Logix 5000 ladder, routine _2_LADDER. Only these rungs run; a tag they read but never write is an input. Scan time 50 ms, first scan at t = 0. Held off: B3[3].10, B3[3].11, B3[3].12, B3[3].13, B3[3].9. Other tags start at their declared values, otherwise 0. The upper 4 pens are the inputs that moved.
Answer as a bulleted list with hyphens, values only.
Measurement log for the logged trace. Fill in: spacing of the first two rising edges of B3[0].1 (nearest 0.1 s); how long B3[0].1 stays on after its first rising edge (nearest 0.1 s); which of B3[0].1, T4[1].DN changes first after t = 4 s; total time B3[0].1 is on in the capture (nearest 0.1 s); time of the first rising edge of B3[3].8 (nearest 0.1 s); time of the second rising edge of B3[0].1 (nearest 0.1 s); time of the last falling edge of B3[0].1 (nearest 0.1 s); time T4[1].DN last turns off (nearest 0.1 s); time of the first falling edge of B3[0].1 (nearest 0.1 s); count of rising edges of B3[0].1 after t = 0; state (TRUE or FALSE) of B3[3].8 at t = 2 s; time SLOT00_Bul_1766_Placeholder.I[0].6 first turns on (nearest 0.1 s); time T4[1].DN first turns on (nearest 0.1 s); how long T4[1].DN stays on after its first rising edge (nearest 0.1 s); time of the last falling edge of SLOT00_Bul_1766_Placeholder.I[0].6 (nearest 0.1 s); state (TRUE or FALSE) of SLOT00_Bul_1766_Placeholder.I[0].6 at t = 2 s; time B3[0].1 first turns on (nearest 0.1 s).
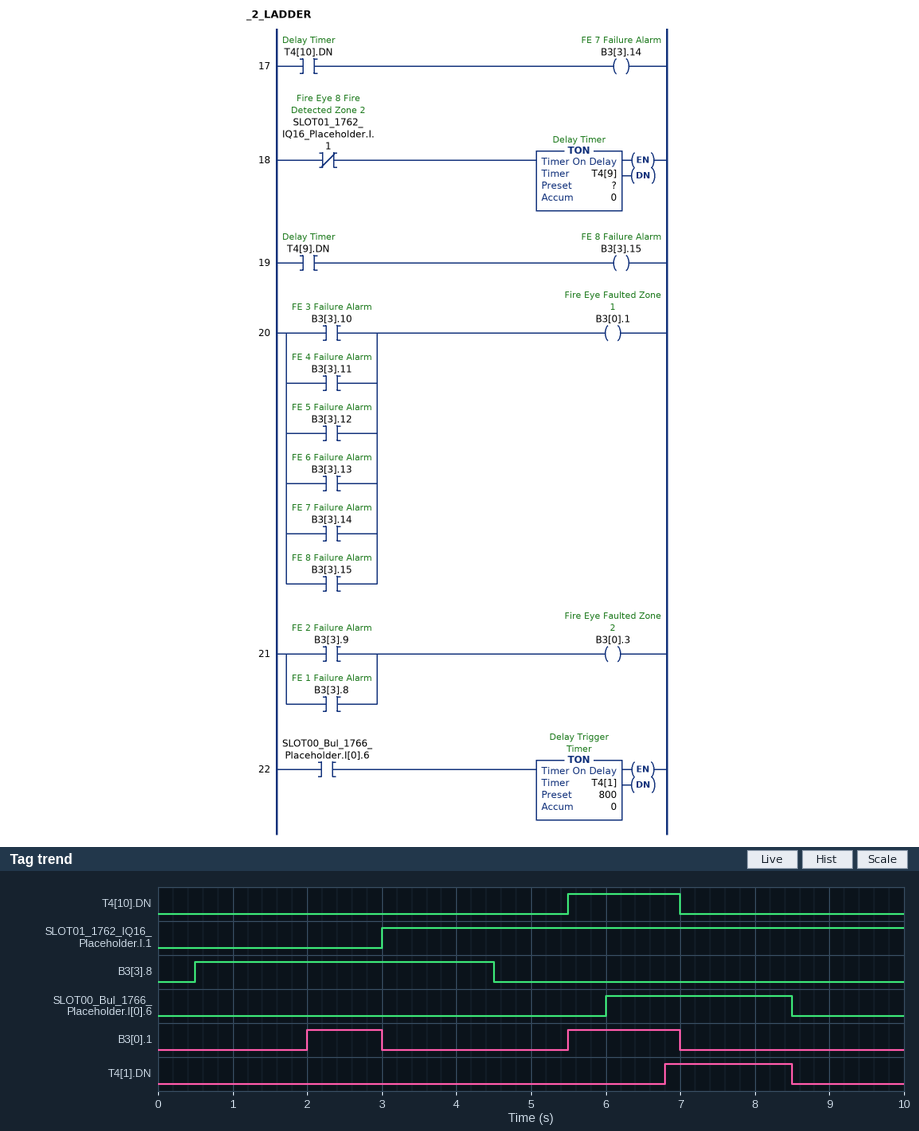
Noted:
- 3.5 s
- 1.0 s
- B3[0].1
- 2.5 s
- 0.5 s
- 5.5 s
- 7.0 s
- 8.5 s
- 3.0 s
- 2
- TRUE
- 6.0 s
- 6.8 s
- 1.7 s
- 8.5 s
- FALSE
- 2.0 s
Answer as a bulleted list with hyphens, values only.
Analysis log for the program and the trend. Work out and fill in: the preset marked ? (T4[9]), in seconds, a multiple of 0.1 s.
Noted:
- 2.0 s
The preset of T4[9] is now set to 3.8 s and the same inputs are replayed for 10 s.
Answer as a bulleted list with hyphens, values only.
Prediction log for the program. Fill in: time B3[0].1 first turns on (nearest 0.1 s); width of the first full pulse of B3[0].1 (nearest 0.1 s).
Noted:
- 5.5 s
- 1.5 s
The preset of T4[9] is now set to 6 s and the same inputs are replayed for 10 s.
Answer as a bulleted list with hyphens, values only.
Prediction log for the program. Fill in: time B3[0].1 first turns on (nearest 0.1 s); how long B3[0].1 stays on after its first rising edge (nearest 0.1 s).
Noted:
- 5.5 s
- 1.5 s
